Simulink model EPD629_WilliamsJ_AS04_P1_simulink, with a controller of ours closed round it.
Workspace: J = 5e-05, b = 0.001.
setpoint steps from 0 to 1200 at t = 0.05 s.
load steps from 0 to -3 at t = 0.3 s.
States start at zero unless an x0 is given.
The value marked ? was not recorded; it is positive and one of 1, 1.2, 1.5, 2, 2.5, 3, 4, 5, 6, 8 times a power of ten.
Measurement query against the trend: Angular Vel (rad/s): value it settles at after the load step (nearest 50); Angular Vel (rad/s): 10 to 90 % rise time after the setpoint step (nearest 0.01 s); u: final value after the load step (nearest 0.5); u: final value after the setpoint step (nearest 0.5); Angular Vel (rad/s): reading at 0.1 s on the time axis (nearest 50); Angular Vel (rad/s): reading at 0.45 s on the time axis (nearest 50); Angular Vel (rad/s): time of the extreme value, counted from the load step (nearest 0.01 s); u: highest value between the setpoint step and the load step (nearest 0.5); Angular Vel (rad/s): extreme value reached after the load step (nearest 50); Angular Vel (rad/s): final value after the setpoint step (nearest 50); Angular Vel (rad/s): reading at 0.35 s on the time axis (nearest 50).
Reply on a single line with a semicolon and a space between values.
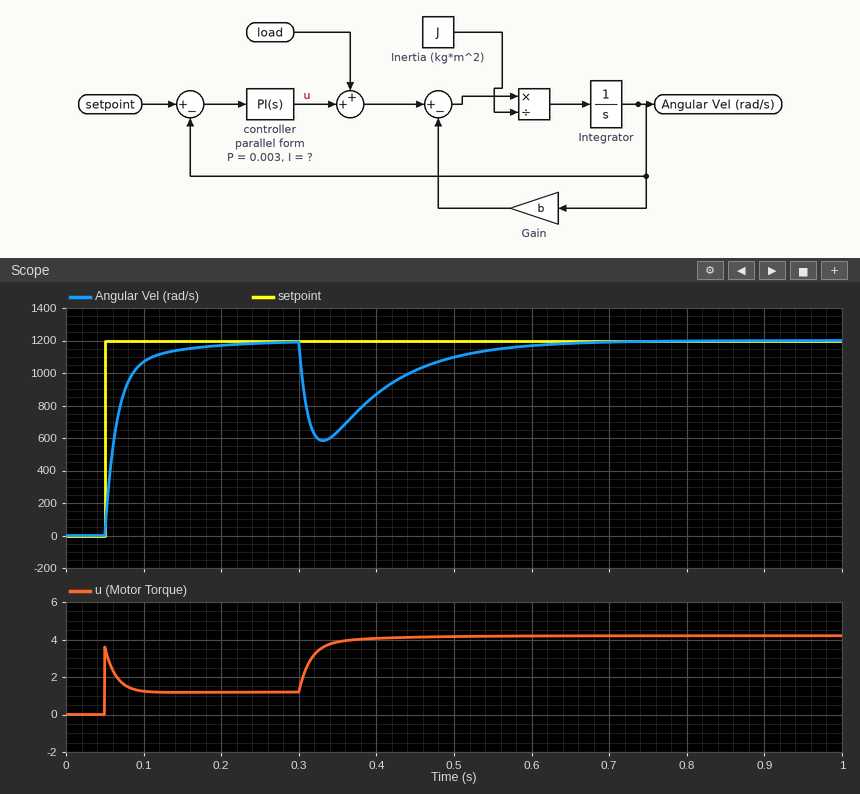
1200; 0.05 s; 4.0; 1.0; 1050; 1000; 0.03 s; 3.5; 600; 1200; 650
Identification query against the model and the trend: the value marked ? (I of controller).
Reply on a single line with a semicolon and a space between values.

0.04
